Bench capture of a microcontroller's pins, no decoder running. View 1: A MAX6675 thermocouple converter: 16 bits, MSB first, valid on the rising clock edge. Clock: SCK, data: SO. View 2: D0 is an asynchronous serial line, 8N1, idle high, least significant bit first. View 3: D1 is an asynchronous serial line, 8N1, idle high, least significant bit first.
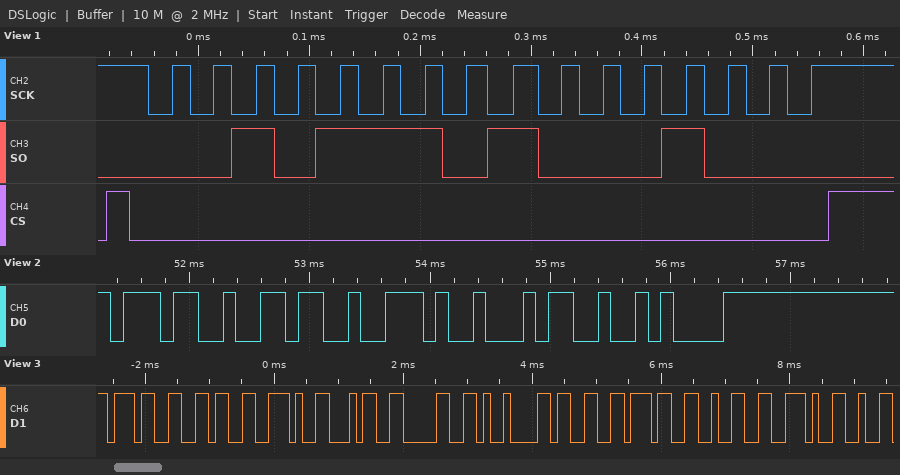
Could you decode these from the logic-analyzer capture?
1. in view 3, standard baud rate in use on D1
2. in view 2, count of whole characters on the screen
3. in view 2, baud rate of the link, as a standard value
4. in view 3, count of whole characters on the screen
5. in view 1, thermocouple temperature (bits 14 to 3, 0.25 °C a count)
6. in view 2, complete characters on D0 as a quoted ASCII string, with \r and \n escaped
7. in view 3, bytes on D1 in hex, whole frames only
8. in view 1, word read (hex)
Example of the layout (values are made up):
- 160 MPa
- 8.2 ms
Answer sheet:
- 9600 baud
- 5
- 9600 baud
- 10
- 372.25 °C
- "76.4\n"
- 37 36 2E 34 30 09 33 37 32 2E
- 0x2E88
